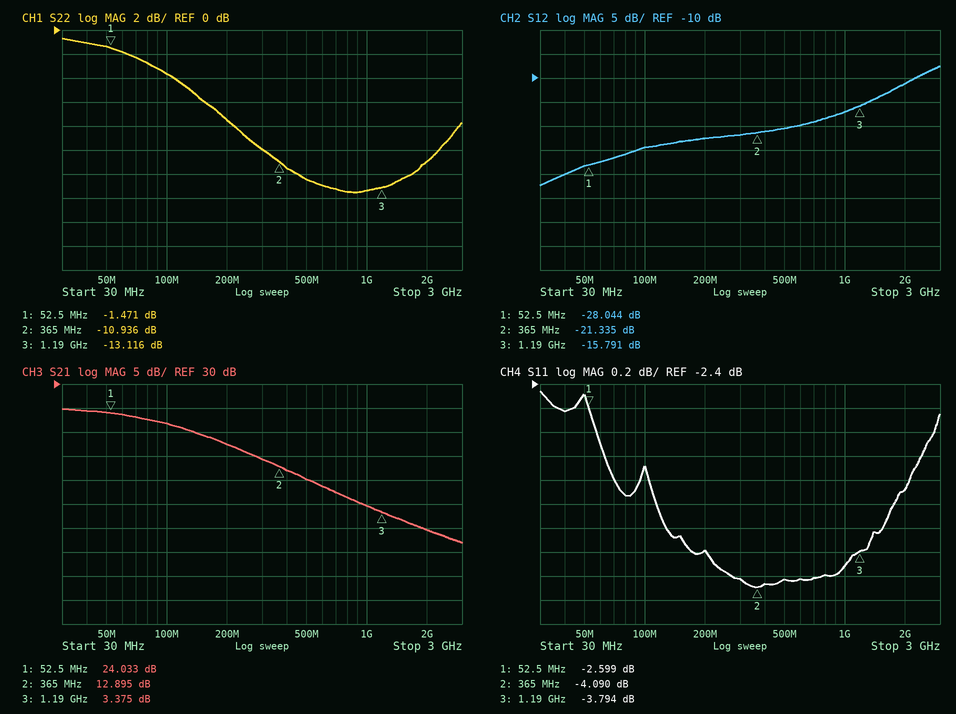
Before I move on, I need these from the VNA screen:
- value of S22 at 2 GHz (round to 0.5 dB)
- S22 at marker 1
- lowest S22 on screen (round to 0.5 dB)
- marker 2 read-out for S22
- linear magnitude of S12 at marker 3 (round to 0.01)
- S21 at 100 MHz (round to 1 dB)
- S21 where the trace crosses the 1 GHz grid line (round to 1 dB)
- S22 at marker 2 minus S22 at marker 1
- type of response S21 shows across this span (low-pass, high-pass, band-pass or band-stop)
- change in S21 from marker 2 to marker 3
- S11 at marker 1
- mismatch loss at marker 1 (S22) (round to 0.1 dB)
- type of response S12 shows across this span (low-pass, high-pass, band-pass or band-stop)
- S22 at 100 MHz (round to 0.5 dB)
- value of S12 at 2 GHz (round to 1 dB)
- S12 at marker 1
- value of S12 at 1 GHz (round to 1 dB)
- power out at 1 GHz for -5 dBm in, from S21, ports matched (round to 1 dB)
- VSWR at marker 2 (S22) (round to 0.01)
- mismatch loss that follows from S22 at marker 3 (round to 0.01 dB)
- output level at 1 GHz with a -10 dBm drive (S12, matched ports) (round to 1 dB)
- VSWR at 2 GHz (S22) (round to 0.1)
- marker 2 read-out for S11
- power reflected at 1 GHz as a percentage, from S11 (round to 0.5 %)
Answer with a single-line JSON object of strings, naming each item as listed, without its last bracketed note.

{"value of S22 at 2 GHz": "-11.0 dB", "S22 at marker 1": "-1.471 dB", "lowest S22 on screen": "-13.5 dB", "marker 2 read-out for S22": "-10.936 dB", "linear magnitude of S12 at marker 3": "0.16", "S21 at 100 MHz": "22 dB", "S21 where the trace crosses the 1 GHz grid line": "5 dB", "S22 at marker 2 minus S22 at marker 1": "-9.465 dB", "type of response S21 shows across this span": "low-pass", "change in S21 from marker 2 to marker 3": "-9.520 dB", "S11 at marker 1": "-2.599 dB", "mismatch loss at marker 1 (S22)": "5.4 dB", "type of response S12 shows across this span": "high-pass", "S22 at 100 MHz": "-3.5 dB", "value of S12 at 2 GHz": "-11 dB", "S12 at marker 1": "-28.044 dB", "value of S12 at 1 GHz": "-17 dB", "power out at 1 GHz for -5 dBm in, from S21, ports matched": "0 dBm", "VSWR at marker 2 (S22)": "1.79", "mismatch loss that follows from S22 at marker 3": "0.22 dB", "output level at 1 GHz with a -10 dBm drive (S12, matched ports)": "-27 dBm", "VSWR at 2 GHz (S22)": "1.8", "marker 2 read-out for S11": "-4.090 dB", "power reflected at 1 GHz as a percentage, from S11": "40.5 %"}
